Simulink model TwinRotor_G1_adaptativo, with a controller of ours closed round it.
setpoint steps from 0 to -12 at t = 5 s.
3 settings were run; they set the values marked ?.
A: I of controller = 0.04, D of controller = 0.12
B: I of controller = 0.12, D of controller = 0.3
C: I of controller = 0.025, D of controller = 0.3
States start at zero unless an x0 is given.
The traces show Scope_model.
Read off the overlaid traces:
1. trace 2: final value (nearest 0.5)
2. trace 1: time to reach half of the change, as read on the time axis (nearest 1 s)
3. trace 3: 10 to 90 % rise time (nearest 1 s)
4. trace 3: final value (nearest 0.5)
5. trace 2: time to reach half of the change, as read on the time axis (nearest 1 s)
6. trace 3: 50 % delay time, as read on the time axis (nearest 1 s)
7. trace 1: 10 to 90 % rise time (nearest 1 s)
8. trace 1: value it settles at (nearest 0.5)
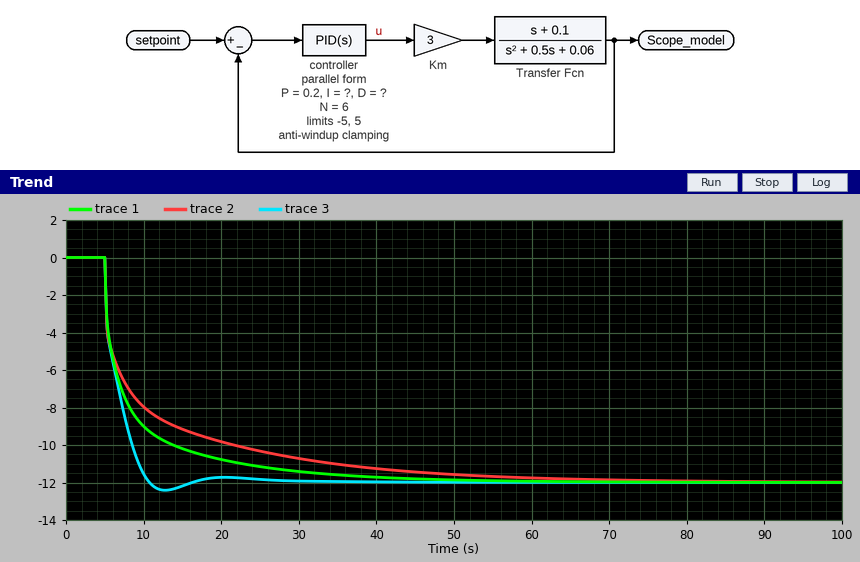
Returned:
-12.0
6 s
4 s
-12.0
7 s
6 s
15 s
-12.0
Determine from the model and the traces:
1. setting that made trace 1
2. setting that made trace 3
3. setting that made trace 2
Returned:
A
B
C
